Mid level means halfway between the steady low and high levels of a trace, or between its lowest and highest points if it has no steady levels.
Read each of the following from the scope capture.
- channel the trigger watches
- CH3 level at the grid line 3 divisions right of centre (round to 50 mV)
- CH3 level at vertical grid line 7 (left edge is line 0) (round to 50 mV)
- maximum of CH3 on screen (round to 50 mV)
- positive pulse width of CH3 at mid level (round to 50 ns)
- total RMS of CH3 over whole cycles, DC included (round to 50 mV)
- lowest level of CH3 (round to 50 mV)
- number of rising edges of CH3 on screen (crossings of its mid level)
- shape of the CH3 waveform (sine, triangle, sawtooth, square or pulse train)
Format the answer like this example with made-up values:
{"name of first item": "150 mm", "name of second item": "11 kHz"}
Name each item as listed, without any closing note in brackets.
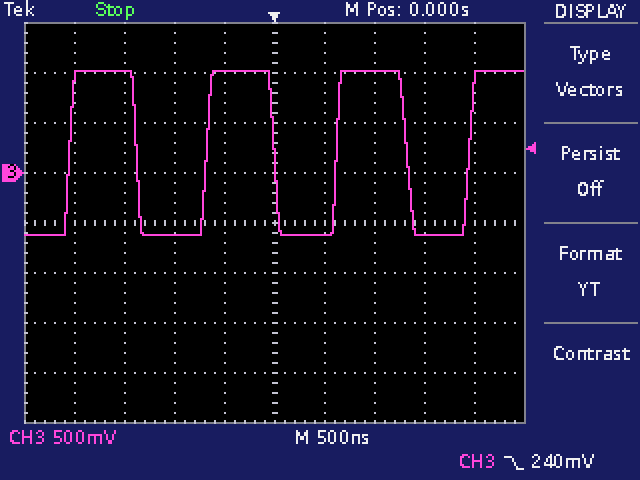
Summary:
{"channel the trigger watches": "CH3", "CH3 level at the grid line 3 divisions right of centre": "-600 mV", "CH3 level at vertical grid line 7 (left edge is line 0)": "1.00 V", "maximum of CH3 on screen": "1.00 V", "positive pulse width of CH3 at mid level": "700 ns", "total RMS of CH3 over whole cycles, DC included": "800 mV", "lowest level of CH3": "-600 mV", "number of rising edges of CH3 on screen": "4", "shape of the CH3 waveform": "square"}
